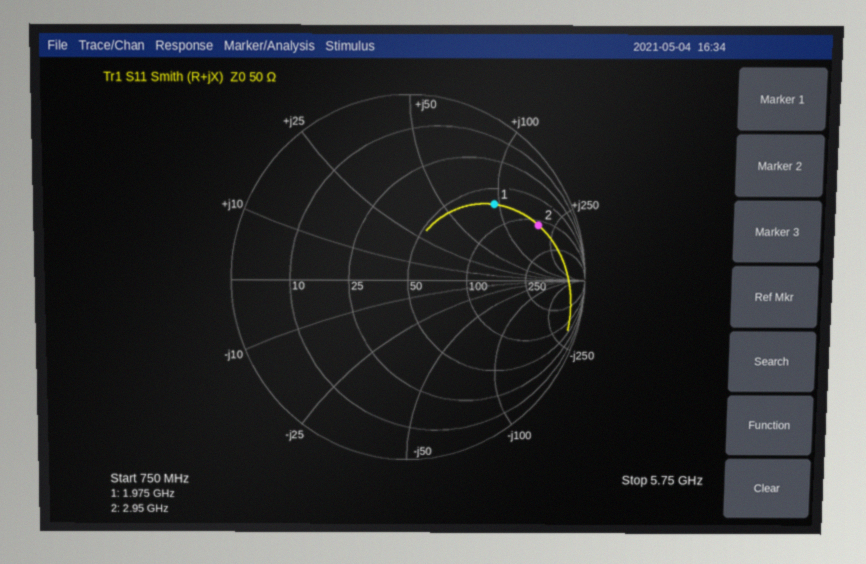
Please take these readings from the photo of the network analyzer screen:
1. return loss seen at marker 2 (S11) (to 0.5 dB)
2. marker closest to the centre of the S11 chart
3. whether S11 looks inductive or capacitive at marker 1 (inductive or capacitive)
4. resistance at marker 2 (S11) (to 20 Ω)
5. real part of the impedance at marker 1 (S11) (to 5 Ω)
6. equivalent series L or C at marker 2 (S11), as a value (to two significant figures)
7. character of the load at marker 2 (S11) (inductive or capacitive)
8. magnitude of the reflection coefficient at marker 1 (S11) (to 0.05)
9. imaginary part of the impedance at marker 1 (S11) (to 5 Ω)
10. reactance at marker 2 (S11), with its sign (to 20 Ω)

2.0 dB
marker 1
inductive
120 Ω
70 Ω
10 nH
inductive
0.65
+95 Ω
+180 Ω
